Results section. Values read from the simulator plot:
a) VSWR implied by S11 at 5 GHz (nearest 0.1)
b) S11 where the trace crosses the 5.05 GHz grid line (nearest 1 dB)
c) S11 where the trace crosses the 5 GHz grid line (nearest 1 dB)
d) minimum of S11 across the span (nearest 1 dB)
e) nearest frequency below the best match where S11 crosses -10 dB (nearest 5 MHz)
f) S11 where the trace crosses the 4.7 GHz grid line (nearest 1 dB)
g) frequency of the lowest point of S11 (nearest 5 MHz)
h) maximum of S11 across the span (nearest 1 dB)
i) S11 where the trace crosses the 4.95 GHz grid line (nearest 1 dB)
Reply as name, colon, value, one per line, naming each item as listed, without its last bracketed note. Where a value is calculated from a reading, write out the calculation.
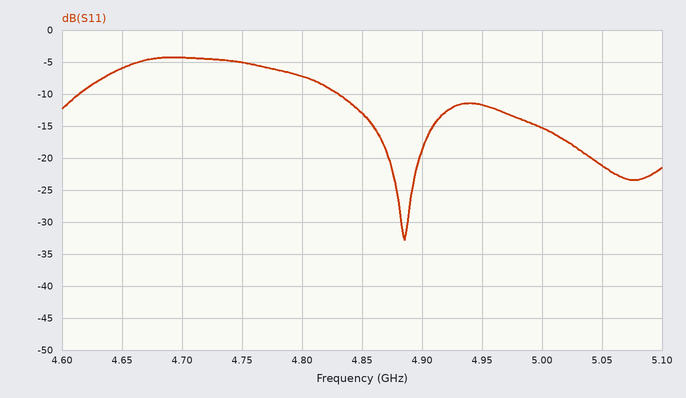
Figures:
VSWR implied by S11 at 5 GHz: |Γ| = 10^(-15/20) = 0.1778; VSWR = (1 + 0.1778)/(1 − 0.1778) ≈ 1.4
S11 where the trace crosses the 5.05 GHz grid line: -21 dB
S11 where the trace crosses the 5 GHz grid line: -15 dB
minimum of S11 across the span: -33 dB
nearest frequency below the best match where S11 crosses -10 dB: 4.830 GHz
S11 where the trace crosses the 4.7 GHz grid line: -4 dB
frequency of the lowest point of S11: 4.885 GHz
maximum of S11 across the span: -4 dB
S11 where the trace crosses the 4.95 GHz grid line: -12 dB
